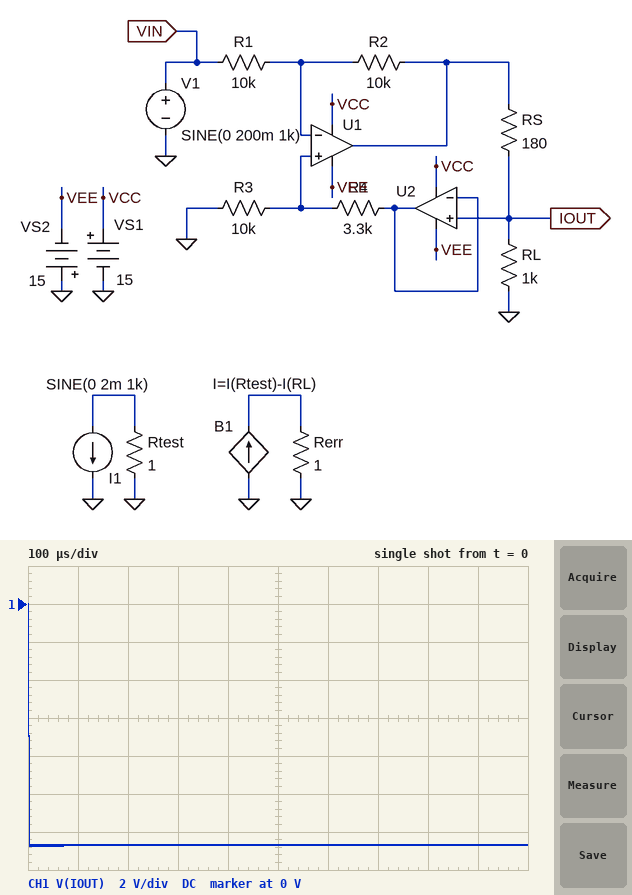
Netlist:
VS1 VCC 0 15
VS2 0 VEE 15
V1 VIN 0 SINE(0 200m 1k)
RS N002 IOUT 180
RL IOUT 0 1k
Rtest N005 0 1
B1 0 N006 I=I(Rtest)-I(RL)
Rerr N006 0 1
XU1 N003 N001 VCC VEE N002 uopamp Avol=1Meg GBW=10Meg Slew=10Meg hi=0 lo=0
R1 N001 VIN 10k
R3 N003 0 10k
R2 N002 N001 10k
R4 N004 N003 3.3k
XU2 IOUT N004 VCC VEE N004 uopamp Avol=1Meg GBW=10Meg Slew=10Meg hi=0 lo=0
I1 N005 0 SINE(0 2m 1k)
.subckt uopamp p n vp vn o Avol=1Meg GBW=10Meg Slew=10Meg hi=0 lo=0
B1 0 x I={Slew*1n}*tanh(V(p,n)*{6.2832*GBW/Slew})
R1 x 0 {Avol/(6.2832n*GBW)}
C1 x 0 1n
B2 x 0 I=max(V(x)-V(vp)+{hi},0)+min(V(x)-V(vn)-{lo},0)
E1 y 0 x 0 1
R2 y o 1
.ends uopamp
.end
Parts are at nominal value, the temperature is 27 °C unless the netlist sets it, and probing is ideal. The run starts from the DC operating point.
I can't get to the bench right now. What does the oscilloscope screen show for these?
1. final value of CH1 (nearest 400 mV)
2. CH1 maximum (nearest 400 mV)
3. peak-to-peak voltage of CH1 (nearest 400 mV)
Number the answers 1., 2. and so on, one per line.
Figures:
1. -12.8 V
2. 0 V
3. 12.8 V
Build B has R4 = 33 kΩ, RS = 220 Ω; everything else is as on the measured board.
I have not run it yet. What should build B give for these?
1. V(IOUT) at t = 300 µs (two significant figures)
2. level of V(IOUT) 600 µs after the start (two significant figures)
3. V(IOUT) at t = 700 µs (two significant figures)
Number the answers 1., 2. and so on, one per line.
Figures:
1. -250 mV
2. 160 mV
3. 250 mV
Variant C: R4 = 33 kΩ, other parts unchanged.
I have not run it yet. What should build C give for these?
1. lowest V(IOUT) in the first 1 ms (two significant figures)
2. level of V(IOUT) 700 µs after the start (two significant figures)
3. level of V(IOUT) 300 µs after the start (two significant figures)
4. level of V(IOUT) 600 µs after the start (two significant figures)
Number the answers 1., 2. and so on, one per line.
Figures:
1. -280 mV
2. 270 mV
3. -270 mV
4. 160 mV
